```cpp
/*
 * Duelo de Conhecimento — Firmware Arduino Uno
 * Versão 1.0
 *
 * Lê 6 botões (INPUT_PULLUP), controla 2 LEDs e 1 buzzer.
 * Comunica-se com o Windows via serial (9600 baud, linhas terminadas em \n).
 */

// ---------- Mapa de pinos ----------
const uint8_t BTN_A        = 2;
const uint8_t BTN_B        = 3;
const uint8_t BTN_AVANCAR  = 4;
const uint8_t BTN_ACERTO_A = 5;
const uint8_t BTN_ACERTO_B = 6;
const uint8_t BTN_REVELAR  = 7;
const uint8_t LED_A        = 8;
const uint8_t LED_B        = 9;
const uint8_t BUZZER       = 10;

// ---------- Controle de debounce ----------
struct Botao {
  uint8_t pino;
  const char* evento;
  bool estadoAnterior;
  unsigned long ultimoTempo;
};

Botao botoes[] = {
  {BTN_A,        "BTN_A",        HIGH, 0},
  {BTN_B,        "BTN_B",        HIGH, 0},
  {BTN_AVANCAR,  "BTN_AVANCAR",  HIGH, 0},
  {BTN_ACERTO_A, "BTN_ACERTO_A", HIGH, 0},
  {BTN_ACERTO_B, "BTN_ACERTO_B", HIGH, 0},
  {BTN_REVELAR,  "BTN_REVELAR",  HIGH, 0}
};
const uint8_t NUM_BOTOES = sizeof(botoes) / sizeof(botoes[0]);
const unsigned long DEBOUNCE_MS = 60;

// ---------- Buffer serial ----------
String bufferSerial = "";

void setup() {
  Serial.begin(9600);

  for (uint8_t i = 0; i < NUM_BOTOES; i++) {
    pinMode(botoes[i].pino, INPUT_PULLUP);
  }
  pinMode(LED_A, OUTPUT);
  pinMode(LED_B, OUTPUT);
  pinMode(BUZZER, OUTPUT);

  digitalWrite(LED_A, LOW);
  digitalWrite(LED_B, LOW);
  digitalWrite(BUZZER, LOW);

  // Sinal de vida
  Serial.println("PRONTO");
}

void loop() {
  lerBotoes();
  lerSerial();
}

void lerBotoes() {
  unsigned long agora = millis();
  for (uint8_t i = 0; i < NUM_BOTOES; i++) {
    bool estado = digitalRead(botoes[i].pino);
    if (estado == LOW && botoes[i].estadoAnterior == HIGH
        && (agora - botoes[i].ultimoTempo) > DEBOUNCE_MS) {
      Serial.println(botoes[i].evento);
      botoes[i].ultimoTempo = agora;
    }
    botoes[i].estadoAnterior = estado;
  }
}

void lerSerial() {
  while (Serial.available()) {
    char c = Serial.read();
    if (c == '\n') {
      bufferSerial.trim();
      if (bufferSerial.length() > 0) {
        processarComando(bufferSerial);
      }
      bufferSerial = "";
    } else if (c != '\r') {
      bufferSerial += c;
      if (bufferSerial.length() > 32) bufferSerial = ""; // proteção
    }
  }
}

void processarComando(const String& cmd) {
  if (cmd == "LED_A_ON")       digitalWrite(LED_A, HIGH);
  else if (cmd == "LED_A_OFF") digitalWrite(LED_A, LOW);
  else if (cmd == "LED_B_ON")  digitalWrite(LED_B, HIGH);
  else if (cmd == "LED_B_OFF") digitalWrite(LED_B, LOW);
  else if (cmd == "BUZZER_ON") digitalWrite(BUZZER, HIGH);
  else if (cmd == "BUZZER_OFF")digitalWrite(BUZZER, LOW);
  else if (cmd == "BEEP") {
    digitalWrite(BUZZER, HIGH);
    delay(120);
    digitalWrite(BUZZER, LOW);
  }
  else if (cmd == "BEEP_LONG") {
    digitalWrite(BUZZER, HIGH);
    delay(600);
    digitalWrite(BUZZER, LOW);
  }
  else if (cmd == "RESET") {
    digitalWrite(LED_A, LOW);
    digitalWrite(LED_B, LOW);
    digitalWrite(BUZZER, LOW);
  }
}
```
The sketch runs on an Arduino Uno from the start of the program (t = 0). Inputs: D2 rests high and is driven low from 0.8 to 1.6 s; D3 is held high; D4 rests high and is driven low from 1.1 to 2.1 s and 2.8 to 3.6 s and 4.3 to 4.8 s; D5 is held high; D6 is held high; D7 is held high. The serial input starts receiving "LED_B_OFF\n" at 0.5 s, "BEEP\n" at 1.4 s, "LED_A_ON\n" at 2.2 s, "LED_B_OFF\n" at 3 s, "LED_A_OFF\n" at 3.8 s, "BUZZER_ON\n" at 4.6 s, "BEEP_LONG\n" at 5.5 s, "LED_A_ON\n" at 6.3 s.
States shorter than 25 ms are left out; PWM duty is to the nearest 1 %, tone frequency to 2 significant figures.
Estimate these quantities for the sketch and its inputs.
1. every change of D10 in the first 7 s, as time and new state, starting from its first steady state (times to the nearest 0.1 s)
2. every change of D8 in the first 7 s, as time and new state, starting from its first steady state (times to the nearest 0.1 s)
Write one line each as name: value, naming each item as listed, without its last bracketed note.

every change of D10 in the first 7 s, as time and new state, starting from its first steady state: 0 s low; 1.4 s high; 1.5 s low; 4.6 s high; 6.1 s low
every change of D8 in the first 7 s, as time and new state, starting from its first steady state: 0 s low; 2.2 s high; 3.8 s low; 6.3 s high
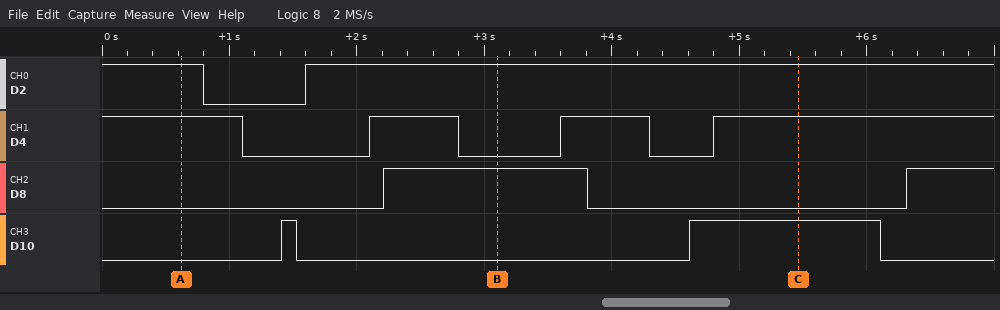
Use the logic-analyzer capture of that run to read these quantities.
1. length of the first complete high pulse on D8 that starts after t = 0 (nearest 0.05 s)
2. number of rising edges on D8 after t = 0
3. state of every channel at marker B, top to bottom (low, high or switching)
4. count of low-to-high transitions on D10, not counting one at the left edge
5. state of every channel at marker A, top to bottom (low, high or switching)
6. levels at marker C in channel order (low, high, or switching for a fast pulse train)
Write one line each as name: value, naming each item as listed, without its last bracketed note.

length of the first complete high pulse on D8 that starts after t = 0: 1.60 s
number of rising edges on D8 after t = 0: 2
state of every channel at marker B, top to bottom: D2 high, D4 low, D8 high, D10 low
count of low-to-high transitions on D10, not counting one at the left edge: 2
state of every channel at marker A, top to bottom: D2 high, D4 high, D8 low, D10 low
levels at marker C in channel order: D2 high, D4 high, D8 low, D10 high
